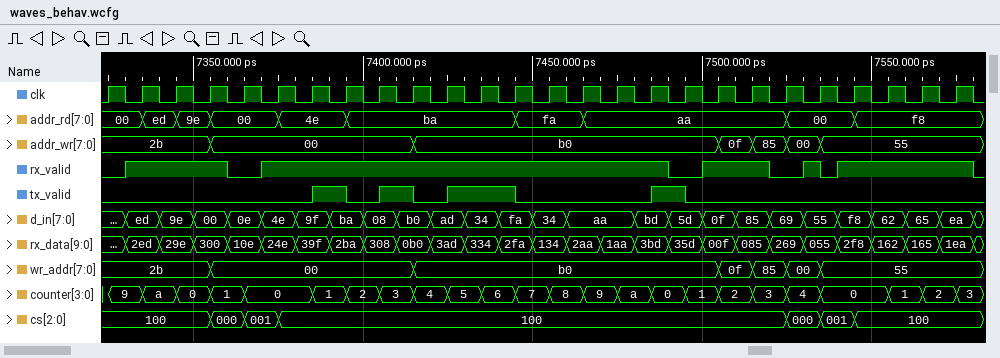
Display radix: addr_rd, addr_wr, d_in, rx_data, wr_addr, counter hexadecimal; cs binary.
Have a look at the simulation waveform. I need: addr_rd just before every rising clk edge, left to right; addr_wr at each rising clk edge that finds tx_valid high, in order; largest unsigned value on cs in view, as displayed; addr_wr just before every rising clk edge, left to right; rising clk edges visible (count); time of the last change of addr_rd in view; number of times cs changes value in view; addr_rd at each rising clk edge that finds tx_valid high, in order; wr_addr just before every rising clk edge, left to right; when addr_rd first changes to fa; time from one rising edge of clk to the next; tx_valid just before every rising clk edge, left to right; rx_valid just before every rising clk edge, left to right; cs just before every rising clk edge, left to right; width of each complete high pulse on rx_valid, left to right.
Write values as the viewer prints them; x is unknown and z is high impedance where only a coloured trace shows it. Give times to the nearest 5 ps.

00, 00, ed, 9e, 00, 00, 4e, 4e, ba, ba, ba, ba, ba, fa, fa, aa, aa, aa, aa, aa, aa, 00, 00, f8, f8, f8
00, 00, b0, b0, b0
100
2b, 2b, 2b, 2b, 00, 00, 00, 00, 00, 00, b0, b0, b0, b0, b0, b0, b0, b0, b0, 0f, 85, 00, 55, 55, 55, 55
26
7545 ps
6
4e, ba, ba, ba, aa
2b, 2b, 2b, 2b, 00, 00, 00, 00, 00, 00, b0, b0, b0, b0, b0, b0, b0, b0, b0, 0f, 85, 00, 55, 55, 55, 55
7445 ps
10 ps
0 0 0 0 0 0 0 1 0 1 0 1 1 0 0 0 0 1 0 0 0 0 0 0 0 0
0 1 1 1 0 1 1 1 1 1 1 1 1 1 1 1 1 0 1 1 0 1 1 1 1 1
100, 100, 100, 100, 000, 001, 100, 100, 100, 100, 100, 100, 100, 100, 100, 100, 100, 100, 100, 100, 100, 000, 001, 100, 100, 100
30 ps, 120 ps, 20 ps, 5 ps, 40 ps
